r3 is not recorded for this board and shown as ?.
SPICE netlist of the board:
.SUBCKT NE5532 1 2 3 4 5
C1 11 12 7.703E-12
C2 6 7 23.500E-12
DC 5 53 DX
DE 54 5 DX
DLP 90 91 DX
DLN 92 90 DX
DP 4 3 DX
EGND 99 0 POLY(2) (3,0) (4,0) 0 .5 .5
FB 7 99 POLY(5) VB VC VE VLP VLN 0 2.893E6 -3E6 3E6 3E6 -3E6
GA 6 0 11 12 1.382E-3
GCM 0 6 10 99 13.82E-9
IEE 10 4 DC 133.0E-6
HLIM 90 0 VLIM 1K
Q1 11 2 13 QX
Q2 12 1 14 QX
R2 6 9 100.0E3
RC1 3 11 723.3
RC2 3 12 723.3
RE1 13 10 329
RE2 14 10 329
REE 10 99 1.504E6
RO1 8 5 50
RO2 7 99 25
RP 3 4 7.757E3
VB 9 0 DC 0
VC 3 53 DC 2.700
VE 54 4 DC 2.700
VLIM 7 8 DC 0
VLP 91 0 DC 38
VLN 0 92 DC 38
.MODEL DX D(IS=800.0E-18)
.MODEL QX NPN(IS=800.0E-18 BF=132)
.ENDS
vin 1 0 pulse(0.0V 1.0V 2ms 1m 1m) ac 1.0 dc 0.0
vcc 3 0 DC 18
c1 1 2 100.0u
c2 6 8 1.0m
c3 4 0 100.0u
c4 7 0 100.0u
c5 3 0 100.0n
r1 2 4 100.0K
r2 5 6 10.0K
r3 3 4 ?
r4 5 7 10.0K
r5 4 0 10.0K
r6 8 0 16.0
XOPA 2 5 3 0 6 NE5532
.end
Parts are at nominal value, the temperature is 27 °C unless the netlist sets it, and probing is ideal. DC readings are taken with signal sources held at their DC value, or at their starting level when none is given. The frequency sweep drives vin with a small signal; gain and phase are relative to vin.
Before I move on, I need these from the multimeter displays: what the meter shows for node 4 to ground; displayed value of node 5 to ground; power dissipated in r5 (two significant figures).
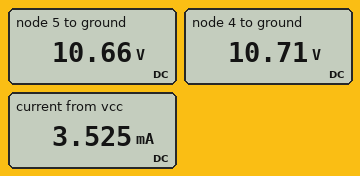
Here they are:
10.71 V
10.66 V
11 mW
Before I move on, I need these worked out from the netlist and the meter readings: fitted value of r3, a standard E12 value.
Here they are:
6.8 kΩ
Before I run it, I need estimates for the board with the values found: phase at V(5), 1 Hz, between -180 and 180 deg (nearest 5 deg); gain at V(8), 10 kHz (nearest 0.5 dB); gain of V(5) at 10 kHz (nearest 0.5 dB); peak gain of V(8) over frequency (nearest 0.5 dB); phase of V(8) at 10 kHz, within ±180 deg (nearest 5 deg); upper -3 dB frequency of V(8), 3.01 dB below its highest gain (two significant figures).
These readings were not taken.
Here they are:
0 deg
6.0 dB
0 dB
6.0 dB
0 deg
1.2 MHz
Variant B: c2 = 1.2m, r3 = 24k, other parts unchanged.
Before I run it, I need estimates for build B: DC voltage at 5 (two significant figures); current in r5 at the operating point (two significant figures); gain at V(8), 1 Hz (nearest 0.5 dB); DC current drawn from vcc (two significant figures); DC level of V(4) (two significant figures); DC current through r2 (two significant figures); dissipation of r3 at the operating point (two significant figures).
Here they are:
5.2 V
530 µA
-12.5 dB
3.0 mA
5.3 V
490 nA
6.7 mW
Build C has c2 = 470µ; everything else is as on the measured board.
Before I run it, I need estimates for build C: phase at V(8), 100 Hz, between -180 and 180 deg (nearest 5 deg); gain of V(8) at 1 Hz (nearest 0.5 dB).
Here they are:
10 deg
-20.5 dB
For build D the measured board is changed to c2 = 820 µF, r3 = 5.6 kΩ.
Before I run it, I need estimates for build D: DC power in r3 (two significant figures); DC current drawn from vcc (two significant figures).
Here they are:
7.5 mW
3.6 mA
